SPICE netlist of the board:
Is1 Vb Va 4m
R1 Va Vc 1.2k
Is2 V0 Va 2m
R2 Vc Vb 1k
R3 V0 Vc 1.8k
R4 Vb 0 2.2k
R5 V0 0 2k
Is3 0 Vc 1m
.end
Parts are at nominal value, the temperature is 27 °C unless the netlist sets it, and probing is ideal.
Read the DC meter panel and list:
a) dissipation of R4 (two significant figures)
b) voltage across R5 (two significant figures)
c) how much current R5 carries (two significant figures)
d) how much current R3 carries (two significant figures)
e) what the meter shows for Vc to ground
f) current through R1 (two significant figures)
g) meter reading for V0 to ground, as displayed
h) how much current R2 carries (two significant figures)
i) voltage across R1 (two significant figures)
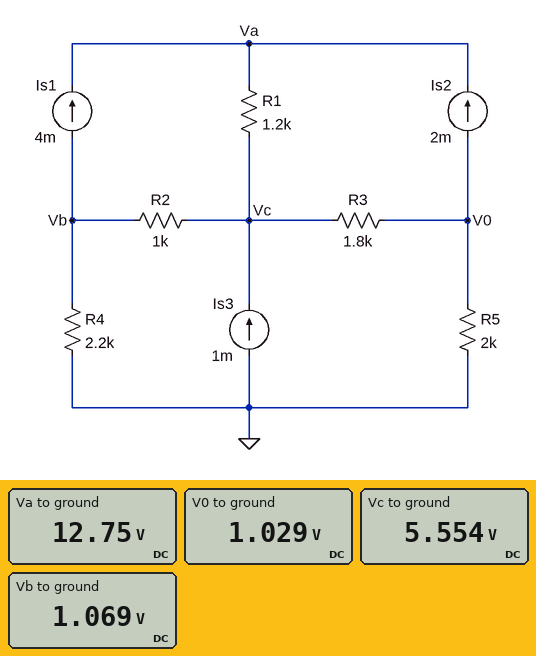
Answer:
520 µW
1.0 V
510 µA
2.5 mA
5.554 V
6.0 mA
1.029 V
4.5 mA
7.2 V
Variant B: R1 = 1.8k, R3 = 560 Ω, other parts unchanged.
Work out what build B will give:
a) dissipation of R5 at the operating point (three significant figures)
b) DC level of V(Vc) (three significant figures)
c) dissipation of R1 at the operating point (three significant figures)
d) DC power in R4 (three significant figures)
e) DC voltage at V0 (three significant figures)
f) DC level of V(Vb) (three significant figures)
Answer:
2.23 mW
3.82 V
64.8 mW
6.79 µW
2.11 V
-122 mV
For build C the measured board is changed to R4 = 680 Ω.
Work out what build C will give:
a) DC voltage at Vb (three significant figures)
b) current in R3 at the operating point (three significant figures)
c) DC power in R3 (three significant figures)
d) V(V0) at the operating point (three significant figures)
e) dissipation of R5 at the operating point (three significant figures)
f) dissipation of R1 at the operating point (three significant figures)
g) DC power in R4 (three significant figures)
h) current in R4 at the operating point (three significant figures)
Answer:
422 mV
2.38 mA
10.2 mW
759 mV
288 µW
43.2 mW
262 µW
620 µA
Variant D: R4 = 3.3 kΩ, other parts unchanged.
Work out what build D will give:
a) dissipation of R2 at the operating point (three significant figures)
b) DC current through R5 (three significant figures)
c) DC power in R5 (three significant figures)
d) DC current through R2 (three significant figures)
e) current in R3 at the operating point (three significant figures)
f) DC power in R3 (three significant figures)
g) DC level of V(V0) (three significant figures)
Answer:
19.5 mW
580 µA
673 µW
4.42 mA
2.58 mA
12.0 mW
1.16 V
